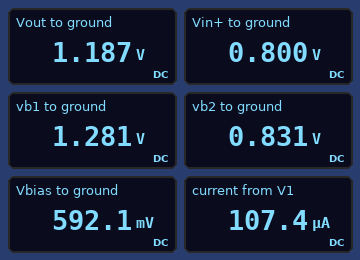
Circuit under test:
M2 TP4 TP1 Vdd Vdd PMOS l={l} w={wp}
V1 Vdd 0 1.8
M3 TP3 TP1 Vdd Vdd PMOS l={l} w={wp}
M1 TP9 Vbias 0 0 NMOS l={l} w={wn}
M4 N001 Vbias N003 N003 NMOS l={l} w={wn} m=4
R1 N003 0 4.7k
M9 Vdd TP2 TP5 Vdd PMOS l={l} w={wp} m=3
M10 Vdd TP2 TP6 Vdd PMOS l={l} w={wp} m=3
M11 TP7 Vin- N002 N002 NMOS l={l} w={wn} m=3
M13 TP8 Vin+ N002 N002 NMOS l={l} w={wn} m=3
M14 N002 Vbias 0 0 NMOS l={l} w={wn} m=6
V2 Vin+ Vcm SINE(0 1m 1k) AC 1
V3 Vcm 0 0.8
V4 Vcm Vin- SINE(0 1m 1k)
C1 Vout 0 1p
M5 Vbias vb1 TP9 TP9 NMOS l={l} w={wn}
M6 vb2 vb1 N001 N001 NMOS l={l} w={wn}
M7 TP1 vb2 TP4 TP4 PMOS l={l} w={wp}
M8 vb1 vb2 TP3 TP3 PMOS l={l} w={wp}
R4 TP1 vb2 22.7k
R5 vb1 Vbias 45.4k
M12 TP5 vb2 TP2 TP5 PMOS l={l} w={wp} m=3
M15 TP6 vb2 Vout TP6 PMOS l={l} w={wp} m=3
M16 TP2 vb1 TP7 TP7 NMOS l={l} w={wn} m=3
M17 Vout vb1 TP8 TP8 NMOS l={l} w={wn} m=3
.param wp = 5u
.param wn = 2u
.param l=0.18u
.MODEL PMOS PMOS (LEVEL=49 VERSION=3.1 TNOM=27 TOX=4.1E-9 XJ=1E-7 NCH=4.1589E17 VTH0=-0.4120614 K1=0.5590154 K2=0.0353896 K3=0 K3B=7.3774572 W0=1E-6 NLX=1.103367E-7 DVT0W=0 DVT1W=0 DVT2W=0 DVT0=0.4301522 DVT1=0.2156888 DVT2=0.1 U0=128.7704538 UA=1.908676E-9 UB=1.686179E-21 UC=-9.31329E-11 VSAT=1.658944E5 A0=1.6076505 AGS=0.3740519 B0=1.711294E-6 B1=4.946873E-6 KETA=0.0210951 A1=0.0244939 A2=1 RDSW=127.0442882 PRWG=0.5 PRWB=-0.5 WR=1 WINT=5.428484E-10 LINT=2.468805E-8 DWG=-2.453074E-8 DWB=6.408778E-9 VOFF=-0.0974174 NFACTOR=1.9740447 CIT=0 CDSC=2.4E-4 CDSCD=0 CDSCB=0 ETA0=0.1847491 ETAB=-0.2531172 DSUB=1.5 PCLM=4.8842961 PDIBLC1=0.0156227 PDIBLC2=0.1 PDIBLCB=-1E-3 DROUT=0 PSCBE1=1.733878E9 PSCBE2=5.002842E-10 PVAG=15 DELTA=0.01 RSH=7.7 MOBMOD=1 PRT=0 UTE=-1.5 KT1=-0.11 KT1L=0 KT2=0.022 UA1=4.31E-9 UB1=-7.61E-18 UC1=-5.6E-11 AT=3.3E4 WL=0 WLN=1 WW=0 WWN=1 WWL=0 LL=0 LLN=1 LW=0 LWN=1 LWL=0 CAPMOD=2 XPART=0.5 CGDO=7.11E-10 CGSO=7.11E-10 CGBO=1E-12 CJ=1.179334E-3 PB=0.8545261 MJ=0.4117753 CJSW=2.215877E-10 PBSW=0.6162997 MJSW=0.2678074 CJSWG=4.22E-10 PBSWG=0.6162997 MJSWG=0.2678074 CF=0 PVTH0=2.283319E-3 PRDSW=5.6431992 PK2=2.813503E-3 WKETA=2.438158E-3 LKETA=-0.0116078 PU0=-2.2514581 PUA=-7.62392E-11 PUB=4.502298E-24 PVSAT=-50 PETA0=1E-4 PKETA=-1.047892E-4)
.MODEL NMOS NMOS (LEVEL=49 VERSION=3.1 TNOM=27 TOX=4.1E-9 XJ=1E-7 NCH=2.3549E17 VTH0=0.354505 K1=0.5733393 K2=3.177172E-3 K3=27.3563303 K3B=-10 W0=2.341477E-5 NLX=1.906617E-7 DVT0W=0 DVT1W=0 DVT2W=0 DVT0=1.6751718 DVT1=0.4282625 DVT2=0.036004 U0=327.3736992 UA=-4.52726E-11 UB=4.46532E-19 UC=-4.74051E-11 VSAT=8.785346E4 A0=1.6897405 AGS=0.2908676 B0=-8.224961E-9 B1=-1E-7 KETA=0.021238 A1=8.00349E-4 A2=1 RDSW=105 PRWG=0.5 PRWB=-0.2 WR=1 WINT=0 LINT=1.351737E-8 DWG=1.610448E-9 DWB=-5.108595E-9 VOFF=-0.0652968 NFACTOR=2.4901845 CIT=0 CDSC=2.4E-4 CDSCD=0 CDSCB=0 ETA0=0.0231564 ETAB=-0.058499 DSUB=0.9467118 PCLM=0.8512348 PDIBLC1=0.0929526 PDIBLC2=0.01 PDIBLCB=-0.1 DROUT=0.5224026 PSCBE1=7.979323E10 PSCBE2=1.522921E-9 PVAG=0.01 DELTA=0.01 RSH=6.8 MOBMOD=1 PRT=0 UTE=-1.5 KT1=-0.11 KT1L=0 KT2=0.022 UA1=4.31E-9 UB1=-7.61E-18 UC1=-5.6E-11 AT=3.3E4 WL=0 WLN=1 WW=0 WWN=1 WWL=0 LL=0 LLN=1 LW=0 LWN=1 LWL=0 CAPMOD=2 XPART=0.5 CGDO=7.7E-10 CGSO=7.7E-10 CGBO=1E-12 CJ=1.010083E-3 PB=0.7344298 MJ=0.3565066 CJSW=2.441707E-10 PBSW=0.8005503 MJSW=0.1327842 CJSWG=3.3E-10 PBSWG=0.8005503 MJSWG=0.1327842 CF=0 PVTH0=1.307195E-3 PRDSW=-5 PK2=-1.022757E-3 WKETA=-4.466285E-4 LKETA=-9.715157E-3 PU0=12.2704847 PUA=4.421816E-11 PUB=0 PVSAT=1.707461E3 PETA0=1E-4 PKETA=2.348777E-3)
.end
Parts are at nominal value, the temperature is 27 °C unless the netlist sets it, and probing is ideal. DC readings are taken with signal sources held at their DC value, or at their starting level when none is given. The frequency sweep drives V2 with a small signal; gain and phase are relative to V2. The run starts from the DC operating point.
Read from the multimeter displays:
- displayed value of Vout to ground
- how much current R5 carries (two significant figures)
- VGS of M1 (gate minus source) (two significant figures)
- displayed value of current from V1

1.187 V
15 µA
590 mV
107.4 µA
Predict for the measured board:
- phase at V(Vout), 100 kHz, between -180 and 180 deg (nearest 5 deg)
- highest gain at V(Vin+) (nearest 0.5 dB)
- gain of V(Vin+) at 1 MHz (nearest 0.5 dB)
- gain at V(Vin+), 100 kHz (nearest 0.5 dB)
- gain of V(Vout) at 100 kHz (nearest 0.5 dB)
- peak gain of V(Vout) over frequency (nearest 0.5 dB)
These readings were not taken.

135 deg
0 dB
0 dB
0 dB
57.5 dB
61.0 dB
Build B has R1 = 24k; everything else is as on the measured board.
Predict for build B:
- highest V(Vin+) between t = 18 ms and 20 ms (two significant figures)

800 mV
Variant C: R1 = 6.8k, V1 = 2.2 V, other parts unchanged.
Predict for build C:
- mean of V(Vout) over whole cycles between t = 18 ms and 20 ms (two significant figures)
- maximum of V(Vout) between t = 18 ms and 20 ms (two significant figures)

1.3 V
2.0 V
